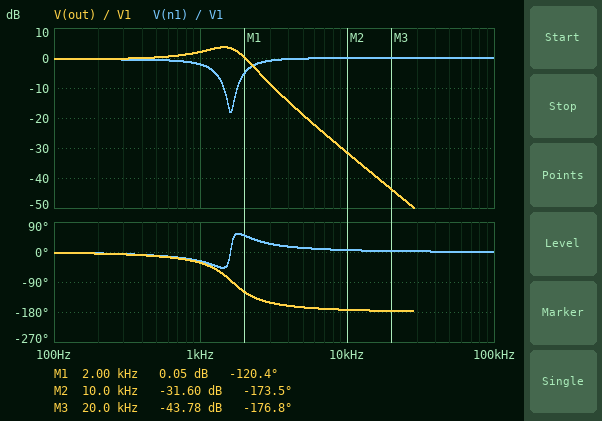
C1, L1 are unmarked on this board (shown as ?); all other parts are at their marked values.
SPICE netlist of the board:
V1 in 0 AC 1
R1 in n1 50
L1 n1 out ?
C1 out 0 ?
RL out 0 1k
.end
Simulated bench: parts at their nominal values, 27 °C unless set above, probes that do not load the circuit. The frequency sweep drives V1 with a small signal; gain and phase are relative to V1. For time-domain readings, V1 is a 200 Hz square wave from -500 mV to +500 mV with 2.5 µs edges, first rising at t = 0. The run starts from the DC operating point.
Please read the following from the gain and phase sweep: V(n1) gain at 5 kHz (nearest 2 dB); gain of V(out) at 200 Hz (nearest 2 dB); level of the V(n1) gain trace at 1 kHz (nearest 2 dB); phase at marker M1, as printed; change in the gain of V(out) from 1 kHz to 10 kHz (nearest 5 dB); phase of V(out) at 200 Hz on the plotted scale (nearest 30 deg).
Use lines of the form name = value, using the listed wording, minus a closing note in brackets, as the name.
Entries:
V(n1) gain at 5 kHz = 0 dB
gain of V(out) at 200 Hz = 0 dB
level of the V(n1) gain trace at 1 kHz = -2 dB
phase at marker M1, as printed = -120.4 deg
change in the gain of V(out) from 1 kHz to 10 kHz = -35 dB
phase of V(out) at 200 Hz on the plotted scale = 0 deg
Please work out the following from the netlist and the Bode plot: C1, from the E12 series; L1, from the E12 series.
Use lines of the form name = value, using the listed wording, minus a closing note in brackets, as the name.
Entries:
C1, from the E12 series = 1.2 µF
L1, from the E12 series = 8.2 mH
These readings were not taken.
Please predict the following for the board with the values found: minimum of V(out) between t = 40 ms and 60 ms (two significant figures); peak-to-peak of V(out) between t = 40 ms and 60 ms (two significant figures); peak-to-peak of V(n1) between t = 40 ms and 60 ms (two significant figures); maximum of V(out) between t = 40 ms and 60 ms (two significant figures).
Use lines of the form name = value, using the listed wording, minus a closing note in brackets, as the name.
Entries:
minimum of V(out) between t = 40 ms and 60 ms = -790 mV
peak-to-peak of V(out) between t = 40 ms and 60 ms = 1.6 V
peak-to-peak of V(n1) between t = 40 ms and 60 ms = 1.2 V
maximum of V(out) between t = 40 ms and 60 ms = 790 mV
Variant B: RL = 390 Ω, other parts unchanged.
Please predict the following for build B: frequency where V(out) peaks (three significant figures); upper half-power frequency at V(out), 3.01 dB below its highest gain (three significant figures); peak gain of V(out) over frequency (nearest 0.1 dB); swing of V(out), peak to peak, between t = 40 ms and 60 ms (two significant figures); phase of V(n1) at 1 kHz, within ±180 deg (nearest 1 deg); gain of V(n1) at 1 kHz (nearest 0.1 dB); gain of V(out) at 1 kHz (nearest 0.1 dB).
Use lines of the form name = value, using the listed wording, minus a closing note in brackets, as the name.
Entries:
frequency where V(out) peaks = 1.43 kHz
upper half-power frequency at V(out), 3.01 dB below its highest gain = 2.03 kHz
peak gain of V(out) over frequency = 1.9 dB
swing of V(out), peak to peak, between t = 40 ms and 60 ms = 1.4 V
phase of V(n1) at 1 kHz, within ±180 deg = -22 deg
gain of V(n1) at 1 kHz = -3.1 dB
gain of V(out) at 1 kHz = 0.9 dB
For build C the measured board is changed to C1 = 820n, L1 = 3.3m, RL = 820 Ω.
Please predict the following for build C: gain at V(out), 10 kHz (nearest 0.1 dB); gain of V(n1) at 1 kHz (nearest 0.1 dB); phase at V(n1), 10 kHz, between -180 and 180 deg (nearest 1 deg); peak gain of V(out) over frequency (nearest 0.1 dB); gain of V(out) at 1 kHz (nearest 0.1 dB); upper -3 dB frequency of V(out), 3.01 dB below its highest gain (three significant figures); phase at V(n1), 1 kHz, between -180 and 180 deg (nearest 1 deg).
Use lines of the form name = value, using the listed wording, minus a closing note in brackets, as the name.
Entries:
gain at V(out), 10 kHz = -20.0 dB
gain of V(n1) at 1 kHz = -0.9 dB
phase at V(n1), 10 kHz, between -180 and 180 deg = 15 deg
peak gain of V(out) over frequency = 1.8 dB
gain of V(out) at 1 kHz = 0 dB
upper -3 dB frequency of V(out), 3.01 dB below its highest gain = 3.74 kHz
phase at V(n1), 1 kHz, between -180 and 180 deg = -15 deg
